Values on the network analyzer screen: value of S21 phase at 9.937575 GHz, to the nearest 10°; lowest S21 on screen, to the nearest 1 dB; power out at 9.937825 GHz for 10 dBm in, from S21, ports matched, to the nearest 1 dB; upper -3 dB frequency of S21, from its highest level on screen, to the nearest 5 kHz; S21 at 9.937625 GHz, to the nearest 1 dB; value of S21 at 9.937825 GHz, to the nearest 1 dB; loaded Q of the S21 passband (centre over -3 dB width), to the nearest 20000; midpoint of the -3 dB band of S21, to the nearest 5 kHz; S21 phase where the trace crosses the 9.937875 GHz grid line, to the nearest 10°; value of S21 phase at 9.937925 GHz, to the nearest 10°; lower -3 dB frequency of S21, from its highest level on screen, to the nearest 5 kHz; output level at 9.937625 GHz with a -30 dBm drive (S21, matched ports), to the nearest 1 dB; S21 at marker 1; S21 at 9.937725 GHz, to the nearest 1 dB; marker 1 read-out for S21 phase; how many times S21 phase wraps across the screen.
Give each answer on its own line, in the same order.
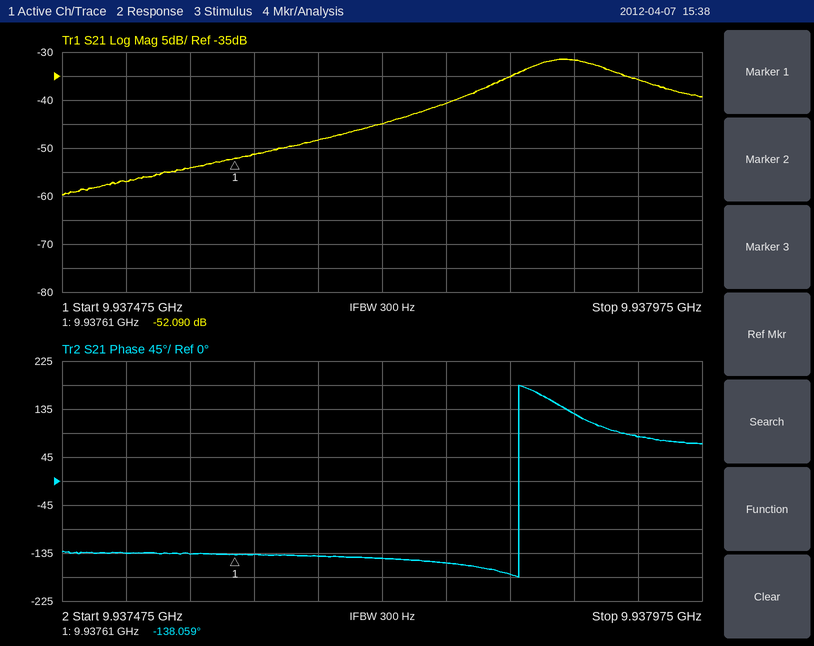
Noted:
-140°
-60 dB
-25 dBm
9.937910 GHz
-51 dB
-35 dB
120000
9.937870 GHz
130°
80°
9.937830 GHz
-81 dBm
-52.090 dB
-45 dB
-138.059°
1
